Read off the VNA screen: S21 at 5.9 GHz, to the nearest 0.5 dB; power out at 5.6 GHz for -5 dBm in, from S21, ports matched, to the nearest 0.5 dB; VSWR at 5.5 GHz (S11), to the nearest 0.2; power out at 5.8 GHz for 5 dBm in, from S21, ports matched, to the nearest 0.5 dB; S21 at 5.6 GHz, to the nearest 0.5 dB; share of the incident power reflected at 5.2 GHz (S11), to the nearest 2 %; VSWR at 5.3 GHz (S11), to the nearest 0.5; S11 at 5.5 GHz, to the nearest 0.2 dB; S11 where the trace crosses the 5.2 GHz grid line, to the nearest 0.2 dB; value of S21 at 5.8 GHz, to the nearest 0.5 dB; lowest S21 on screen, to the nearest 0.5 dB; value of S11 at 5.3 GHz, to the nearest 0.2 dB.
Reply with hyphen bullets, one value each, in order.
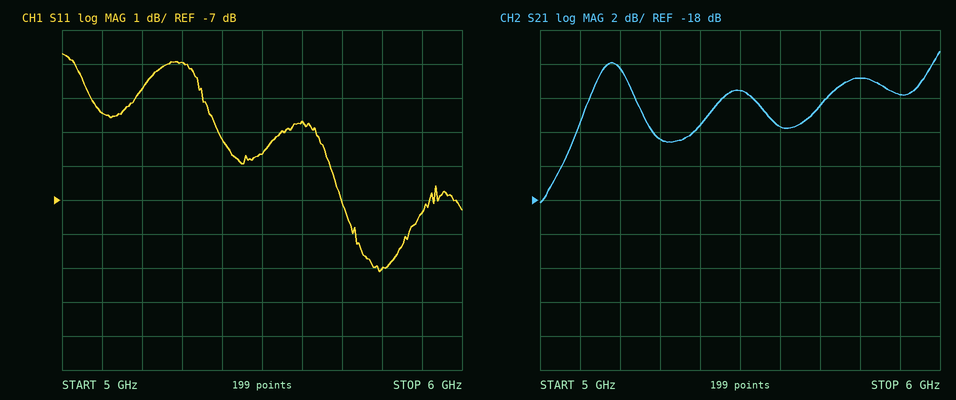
- -12.0 dB
- -18.5 dBm
- 3.2
- -6.0 dBm
- -13.5 dB
- 42 %
- 6.0
- -5.6 dB
- -3.8 dB
- -11.0 dB
- -18.0 dB
- -3.0 dB
